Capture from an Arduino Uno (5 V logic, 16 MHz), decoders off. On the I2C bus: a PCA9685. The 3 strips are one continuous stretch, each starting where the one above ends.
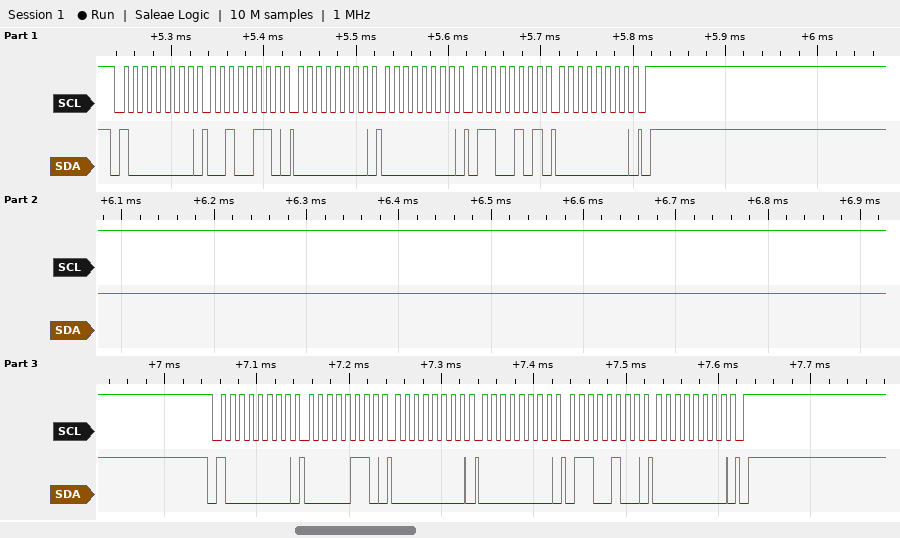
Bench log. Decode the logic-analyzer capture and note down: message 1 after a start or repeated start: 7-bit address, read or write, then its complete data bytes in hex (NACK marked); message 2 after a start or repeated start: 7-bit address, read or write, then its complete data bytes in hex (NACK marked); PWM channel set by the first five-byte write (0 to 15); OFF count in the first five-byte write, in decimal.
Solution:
0x40 write: 26 00 00 65 00
0x40 write: 06 00 00 64 00
8
101
